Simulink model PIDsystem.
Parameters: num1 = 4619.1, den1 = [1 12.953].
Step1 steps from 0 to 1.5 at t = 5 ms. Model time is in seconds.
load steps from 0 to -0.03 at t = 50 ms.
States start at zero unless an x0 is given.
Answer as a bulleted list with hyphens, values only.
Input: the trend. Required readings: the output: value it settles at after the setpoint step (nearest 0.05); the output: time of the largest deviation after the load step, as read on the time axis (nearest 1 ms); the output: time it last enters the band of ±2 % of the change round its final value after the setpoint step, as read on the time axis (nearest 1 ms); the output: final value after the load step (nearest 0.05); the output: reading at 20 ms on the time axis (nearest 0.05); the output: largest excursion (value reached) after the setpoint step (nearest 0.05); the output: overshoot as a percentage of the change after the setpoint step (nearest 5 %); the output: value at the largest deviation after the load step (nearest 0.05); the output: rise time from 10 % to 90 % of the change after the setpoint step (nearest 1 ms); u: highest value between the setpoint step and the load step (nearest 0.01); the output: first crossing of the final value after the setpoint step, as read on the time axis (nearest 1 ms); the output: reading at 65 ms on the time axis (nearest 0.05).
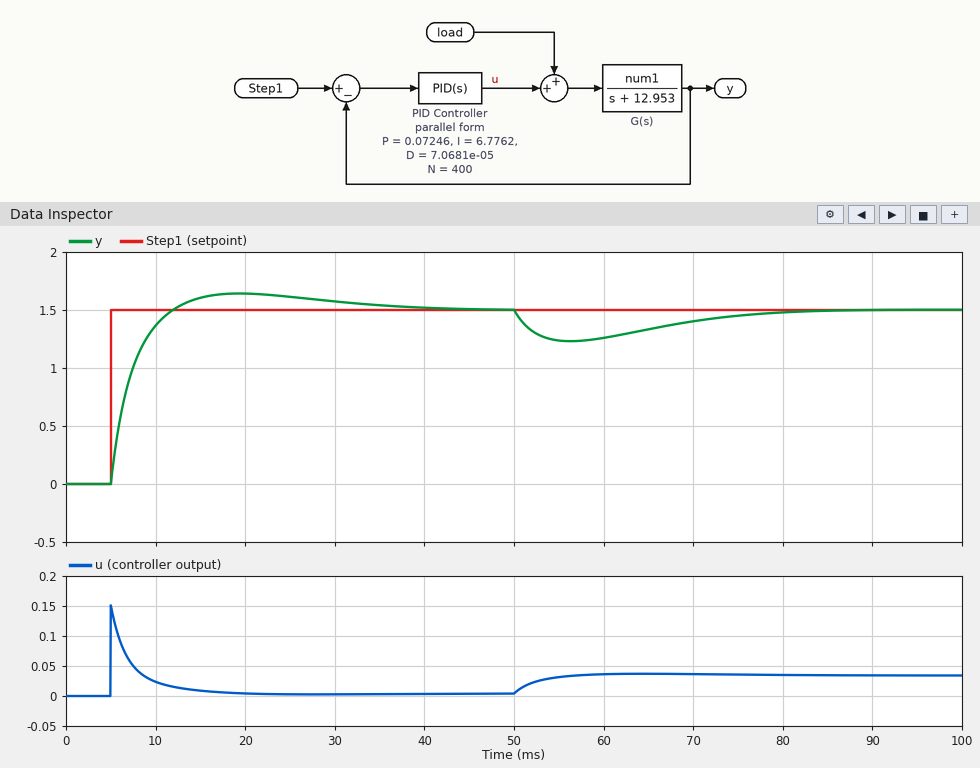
- 1.50
- 56 ms
- 37 ms
- 1.50
- 1.65
- 1.65
- 10 %
- 1.25
- 5 ms
- 0.15
- 12 ms
- 1.35
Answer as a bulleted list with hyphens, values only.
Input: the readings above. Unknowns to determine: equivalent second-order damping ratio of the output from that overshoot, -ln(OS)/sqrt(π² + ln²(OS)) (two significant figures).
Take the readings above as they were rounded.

- 0.59
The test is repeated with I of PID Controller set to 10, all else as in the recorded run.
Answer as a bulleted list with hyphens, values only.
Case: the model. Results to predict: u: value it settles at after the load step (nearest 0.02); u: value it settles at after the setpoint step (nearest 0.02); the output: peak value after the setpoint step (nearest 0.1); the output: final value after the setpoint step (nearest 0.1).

- 0.04
- 0.00
- 1.7
- 1.5
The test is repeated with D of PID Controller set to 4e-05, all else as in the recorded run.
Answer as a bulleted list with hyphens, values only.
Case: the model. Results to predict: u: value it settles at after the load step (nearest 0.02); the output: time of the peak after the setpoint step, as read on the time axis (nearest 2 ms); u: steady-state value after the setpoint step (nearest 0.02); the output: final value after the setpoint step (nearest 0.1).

- 0.04
- 18 ms
- 0.00
- 1.5
